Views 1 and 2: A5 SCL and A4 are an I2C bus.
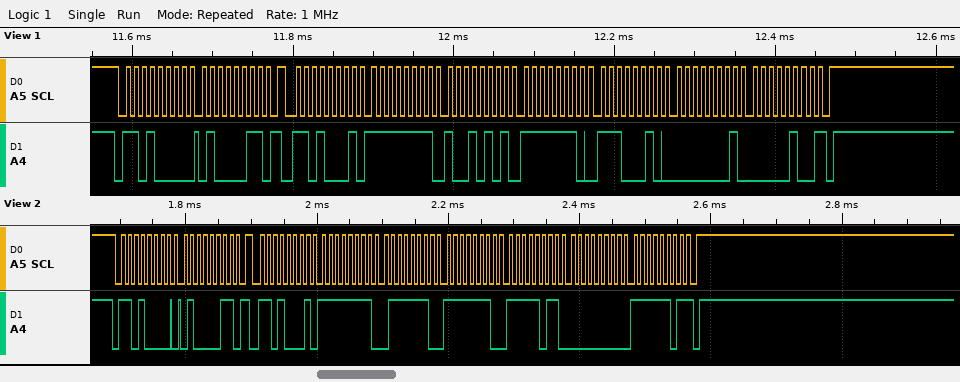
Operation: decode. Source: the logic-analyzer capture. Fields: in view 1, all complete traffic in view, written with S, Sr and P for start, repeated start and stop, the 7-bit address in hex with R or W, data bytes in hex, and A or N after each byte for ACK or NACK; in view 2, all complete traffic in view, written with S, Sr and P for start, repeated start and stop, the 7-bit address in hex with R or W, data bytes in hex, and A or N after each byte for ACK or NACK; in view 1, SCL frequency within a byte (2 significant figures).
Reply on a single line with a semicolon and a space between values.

S 68W A 43 A Sr 68R A FF A 95 A FE A E2 A 01 A 04 N P; S 68W A 43 A Sr 68R A FF A 7E A FE A FB A 00 A FD N P; 100 kHz
